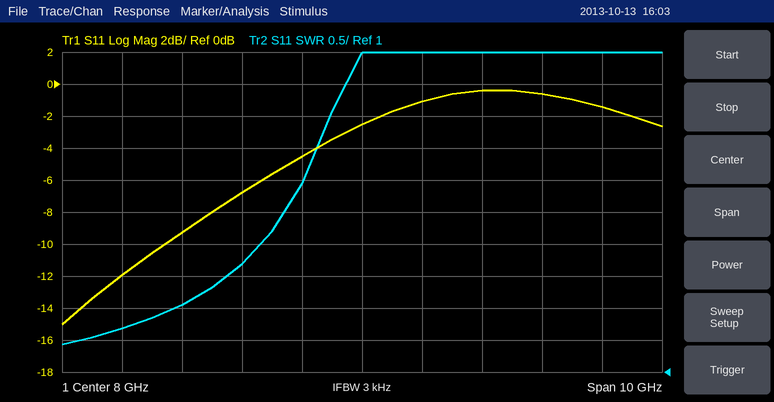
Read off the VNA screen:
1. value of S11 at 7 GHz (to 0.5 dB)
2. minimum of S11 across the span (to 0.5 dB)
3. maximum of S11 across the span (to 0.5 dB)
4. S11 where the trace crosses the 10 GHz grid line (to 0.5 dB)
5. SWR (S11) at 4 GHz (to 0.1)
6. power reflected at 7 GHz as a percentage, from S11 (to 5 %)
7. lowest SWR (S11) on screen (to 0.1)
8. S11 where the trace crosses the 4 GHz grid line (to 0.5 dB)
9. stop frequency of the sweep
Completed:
-4.5 dB
-15.0 dB
-0.5 dB
-0.5 dB
1.7
35 %
1.4
-12.0 dB
13 GHz
